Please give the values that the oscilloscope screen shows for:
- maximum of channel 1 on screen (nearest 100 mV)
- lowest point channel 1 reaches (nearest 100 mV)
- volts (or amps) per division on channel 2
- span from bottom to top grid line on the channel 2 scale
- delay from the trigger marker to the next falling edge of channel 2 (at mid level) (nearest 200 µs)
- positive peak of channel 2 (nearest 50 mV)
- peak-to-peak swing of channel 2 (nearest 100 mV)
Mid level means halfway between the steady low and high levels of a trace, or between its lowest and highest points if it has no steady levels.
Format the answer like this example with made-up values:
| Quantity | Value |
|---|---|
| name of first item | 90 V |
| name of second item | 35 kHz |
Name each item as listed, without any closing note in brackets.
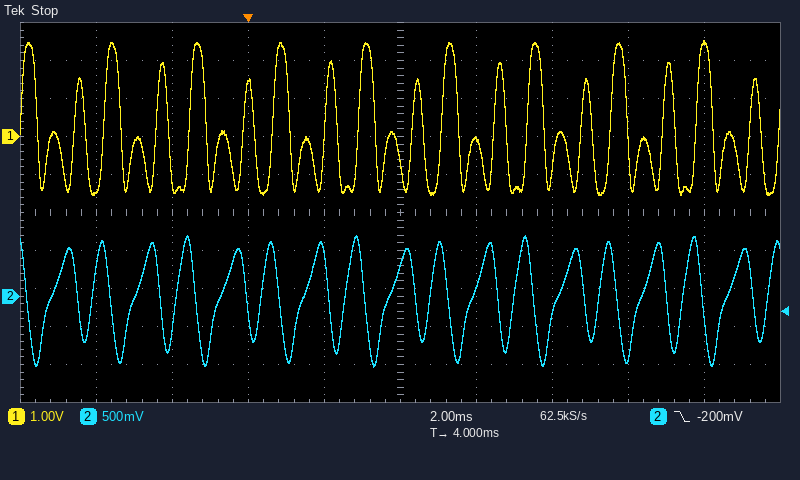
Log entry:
| Quantity | Value |
|---|---|
| maximum of channel 1 on screen | 2.5 V |
| lowest point channel 1 reaches | -1.5 V |
| volts (or amps) per division on channel 2 | 500 mV |
| span from bottom to top grid line on the channel 2 scale | 5 V |
| delay from the trigger marker to the next falling edge of channel 2 (at mid level) | 800 µs |
| positive peak of channel 2 | 800 mV |
| peak-to-peak swing of channel 2 | 1.70 V |
